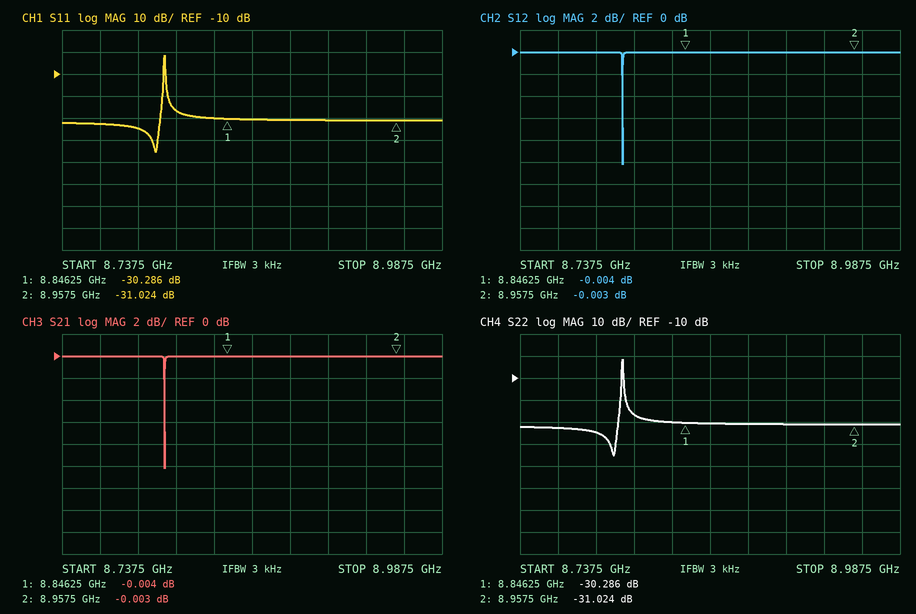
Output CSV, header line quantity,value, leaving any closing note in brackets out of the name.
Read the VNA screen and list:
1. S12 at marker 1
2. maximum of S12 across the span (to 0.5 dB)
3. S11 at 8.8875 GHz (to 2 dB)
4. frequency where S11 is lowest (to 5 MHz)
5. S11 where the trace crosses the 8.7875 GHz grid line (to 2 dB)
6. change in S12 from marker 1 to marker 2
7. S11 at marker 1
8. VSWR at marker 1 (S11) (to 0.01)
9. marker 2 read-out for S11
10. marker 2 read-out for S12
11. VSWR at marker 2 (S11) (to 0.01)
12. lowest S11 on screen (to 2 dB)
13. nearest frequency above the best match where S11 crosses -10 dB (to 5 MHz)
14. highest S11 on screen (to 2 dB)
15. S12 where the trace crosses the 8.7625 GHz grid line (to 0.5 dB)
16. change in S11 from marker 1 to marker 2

quantity,value
S12 at marker 1,-0.004 dB
maximum of S12 across the span,0.0 dB
S11 at 8.8875 GHz,-30 dB
frequency where S11 is lowest,8.800 GHz
S11 where the trace crosses the 8.7875 GHz grid line,-34 dB
change in S12 from marker 1 to marker 2,0.001 dB
S11 at marker 1,-30.286 dB
VSWR at marker 1 (S11),1.06
marker 2 read-out for S11,-31.024 dB
marker 2 read-out for S12,-0.003 dB
VSWR at marker 2 (S11),1.06
lowest S11 on screen,-46 dB
nearest frequency above the best match where S11 crosses -10 dB,8.805 GHz
highest S11 on screen,-2 dB
S12 where the trace crosses the 8.7625 GHz grid line,0.0 dB
change in S11 from marker 1 to marker 2,-0.738 dB
